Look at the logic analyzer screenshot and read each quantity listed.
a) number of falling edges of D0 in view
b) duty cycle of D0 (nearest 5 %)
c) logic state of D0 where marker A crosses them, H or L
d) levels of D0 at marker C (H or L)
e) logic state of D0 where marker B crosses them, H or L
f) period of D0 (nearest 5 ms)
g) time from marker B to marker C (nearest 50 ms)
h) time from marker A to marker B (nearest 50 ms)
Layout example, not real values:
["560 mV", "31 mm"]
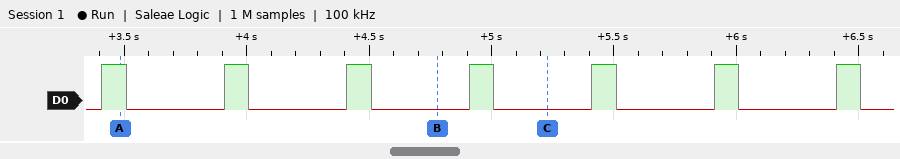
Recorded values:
["7", "20 %", "D0=H", "D0=L", "D0=L", "500 ms", "450 ms", "1300 ms"]
